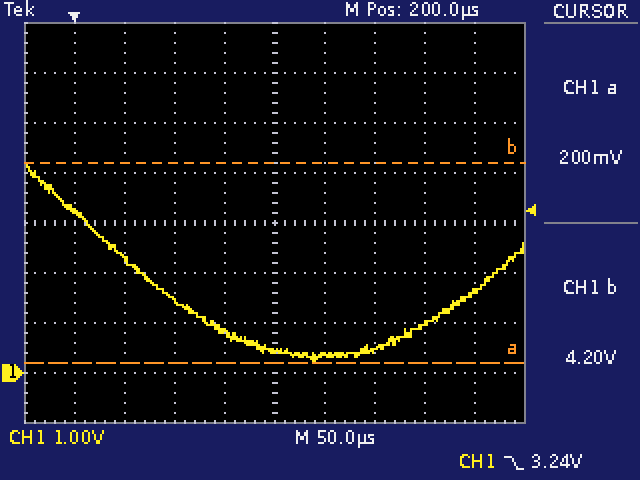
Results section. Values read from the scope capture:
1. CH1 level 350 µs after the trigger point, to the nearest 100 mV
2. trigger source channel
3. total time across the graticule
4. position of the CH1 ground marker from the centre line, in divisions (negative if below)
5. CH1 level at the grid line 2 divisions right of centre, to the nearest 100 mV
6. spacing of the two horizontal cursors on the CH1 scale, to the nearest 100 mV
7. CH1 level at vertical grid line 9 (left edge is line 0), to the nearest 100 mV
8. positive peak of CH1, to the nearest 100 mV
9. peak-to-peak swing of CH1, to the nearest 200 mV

1.0 V
CH1
500 µs
-3.0 div
500 mV
4.0 V
1.6 V
4.2 V
4.0 V
